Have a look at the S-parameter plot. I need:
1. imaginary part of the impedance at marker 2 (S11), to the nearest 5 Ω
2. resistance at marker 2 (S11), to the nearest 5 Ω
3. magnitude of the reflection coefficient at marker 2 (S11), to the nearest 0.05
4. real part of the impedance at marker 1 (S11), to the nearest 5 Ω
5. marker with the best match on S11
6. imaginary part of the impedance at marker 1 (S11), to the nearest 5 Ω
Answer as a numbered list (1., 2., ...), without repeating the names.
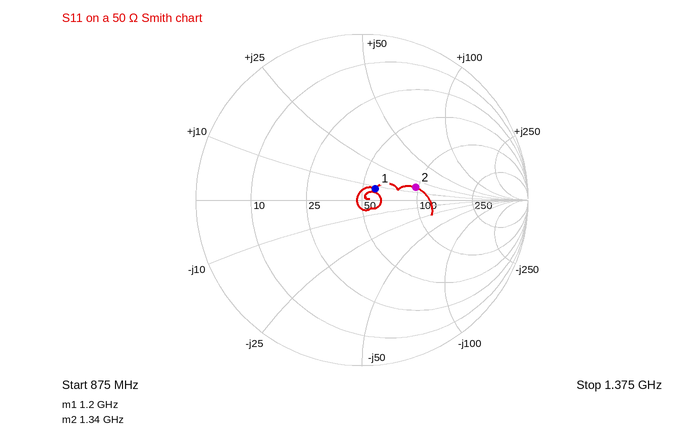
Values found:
1. +15 Ω
2. 95 Ω
3. 0.35
4. 60 Ω
5. marker 1
6. +10 Ω
